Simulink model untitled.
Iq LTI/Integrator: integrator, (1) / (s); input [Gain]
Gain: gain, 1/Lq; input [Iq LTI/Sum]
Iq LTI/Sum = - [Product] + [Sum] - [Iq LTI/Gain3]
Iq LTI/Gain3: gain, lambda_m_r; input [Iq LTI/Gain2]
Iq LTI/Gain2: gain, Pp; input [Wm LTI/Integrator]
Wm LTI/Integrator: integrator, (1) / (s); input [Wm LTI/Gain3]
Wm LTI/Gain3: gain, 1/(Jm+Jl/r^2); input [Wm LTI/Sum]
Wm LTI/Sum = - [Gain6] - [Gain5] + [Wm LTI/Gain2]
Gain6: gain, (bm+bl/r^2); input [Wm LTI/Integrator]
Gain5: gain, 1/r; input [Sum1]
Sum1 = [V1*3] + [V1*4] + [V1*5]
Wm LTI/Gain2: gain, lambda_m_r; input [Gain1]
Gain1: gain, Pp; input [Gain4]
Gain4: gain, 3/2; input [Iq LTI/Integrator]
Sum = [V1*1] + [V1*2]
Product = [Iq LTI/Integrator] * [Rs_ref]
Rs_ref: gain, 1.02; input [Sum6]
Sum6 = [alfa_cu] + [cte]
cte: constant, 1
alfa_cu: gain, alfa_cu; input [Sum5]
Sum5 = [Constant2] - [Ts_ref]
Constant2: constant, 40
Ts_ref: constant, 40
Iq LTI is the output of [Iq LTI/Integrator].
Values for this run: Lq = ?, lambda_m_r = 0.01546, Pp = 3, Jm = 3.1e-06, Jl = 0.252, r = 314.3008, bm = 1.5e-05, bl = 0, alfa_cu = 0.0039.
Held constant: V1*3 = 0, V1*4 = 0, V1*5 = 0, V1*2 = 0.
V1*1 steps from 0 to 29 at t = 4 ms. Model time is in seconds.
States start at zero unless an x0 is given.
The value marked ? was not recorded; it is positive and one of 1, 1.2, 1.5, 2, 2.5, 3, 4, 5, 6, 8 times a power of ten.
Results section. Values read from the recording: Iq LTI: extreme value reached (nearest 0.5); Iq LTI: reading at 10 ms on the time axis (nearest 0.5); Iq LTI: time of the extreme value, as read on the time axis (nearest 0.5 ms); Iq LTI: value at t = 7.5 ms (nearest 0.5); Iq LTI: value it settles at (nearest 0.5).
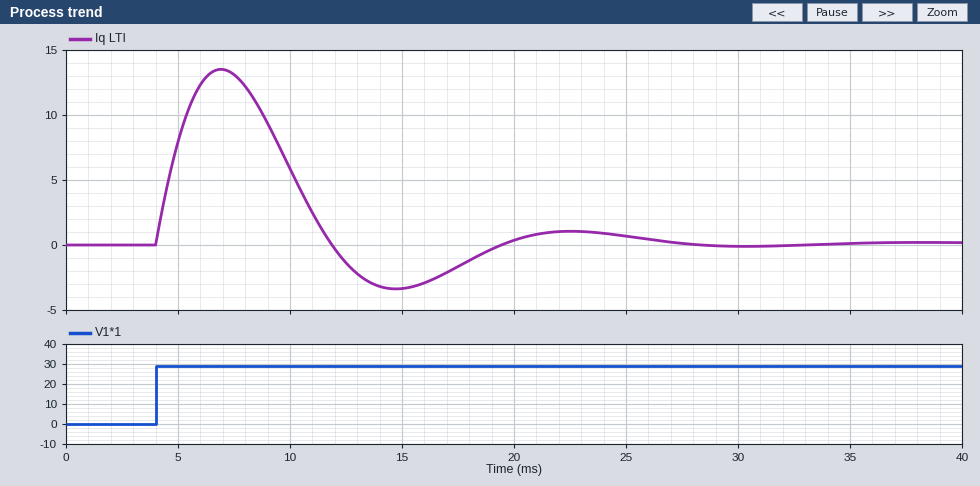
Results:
13.5
6.0
7.0 ms
13.0
0.0
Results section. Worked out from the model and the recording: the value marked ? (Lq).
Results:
0.003
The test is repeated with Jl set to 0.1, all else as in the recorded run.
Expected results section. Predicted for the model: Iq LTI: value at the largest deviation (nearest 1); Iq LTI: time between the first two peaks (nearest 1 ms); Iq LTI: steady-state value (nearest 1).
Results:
12
13 ms
0
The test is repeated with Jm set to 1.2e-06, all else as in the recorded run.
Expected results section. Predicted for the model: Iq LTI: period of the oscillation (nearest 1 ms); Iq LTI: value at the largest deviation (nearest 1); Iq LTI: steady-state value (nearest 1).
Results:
12 ms
12
0
